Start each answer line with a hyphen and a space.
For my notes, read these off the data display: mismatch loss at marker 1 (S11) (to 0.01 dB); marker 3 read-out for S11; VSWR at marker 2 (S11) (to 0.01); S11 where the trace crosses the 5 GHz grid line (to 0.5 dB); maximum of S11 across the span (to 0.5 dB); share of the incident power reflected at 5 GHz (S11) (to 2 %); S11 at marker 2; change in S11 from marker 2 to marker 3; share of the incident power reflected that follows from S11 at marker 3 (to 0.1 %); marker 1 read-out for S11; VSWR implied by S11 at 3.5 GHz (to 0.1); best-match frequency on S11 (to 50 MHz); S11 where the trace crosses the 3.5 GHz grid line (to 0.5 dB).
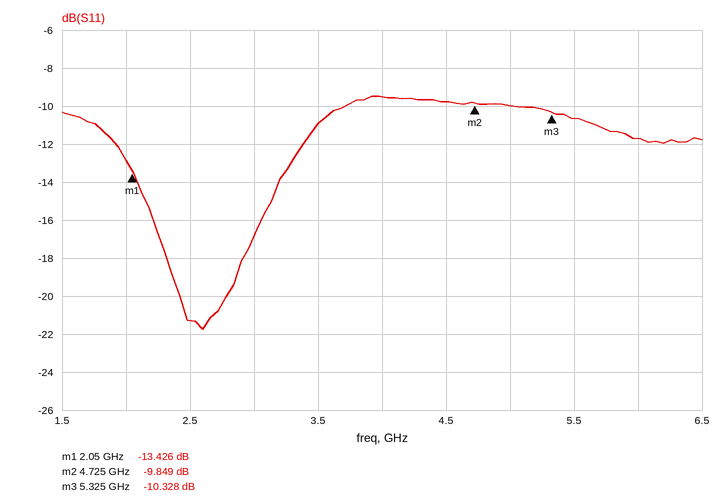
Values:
- 0.20 dB
- -10.328 dB
- 1.95
- -10.0 dB
- -9.5 dB
- 10 %
- -9.849 dB
- -0.479 dB
- 9.3 %
- -13.426 dB
- 1.8
- 2.60 GHz
- -11.0 dB
